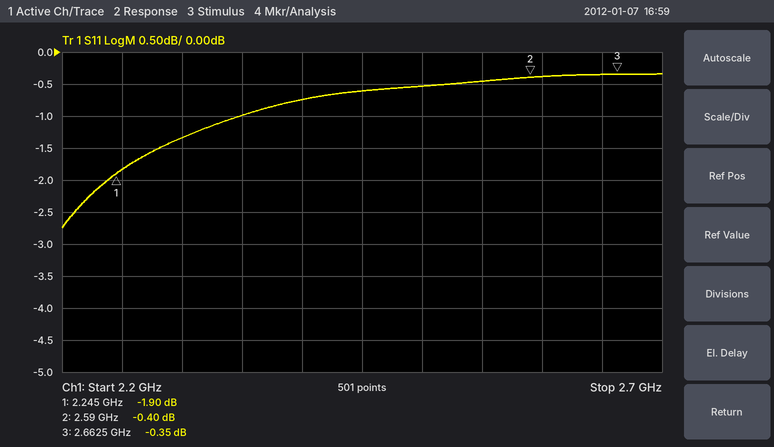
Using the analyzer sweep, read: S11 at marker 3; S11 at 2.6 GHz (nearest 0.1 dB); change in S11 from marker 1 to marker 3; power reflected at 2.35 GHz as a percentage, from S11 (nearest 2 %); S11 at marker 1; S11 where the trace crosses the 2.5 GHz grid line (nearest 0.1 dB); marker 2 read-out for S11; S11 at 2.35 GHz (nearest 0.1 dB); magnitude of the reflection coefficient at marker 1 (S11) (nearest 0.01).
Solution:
-0.35 dB
-0.4 dB
1.55 dB
80 %
-1.90 dB
-0.5 dB
-0.40 dB
-1.0 dB
0.80
